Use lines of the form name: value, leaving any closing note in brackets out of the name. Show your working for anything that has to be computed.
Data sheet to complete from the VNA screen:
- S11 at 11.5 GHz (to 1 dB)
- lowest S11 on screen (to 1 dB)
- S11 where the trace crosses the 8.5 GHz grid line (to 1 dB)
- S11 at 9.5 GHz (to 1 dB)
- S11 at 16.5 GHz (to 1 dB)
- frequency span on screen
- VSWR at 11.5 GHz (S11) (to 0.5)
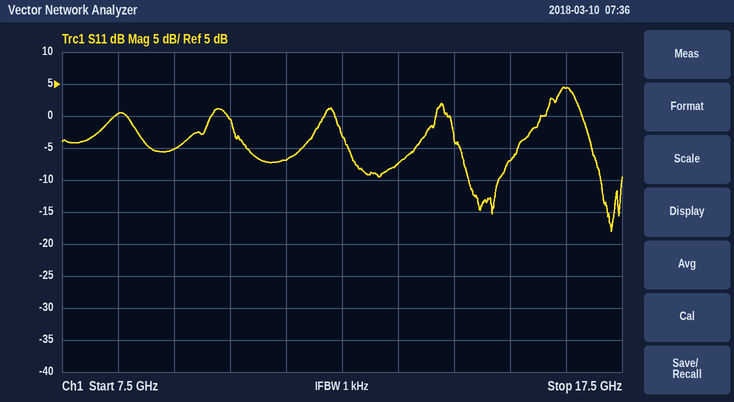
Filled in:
S11 at 11.5 GHz: -7 dB
lowest S11 on screen: -18 dB
S11 where the trace crosses the 8.5 GHz grid line: 0 dB
S11 at 9.5 GHz: -5 dB
S11 at 16.5 GHz: 4 dB
frequency span on screen: 10 GHz
VSWR at 11.5 GHz (S11): |Γ| = 10^(-7/20) = 0.4467; VSWR = (1 + 0.4467)/(1 − 0.4467) ≈ 2.61, so 2.5 to the nearest 0.5
